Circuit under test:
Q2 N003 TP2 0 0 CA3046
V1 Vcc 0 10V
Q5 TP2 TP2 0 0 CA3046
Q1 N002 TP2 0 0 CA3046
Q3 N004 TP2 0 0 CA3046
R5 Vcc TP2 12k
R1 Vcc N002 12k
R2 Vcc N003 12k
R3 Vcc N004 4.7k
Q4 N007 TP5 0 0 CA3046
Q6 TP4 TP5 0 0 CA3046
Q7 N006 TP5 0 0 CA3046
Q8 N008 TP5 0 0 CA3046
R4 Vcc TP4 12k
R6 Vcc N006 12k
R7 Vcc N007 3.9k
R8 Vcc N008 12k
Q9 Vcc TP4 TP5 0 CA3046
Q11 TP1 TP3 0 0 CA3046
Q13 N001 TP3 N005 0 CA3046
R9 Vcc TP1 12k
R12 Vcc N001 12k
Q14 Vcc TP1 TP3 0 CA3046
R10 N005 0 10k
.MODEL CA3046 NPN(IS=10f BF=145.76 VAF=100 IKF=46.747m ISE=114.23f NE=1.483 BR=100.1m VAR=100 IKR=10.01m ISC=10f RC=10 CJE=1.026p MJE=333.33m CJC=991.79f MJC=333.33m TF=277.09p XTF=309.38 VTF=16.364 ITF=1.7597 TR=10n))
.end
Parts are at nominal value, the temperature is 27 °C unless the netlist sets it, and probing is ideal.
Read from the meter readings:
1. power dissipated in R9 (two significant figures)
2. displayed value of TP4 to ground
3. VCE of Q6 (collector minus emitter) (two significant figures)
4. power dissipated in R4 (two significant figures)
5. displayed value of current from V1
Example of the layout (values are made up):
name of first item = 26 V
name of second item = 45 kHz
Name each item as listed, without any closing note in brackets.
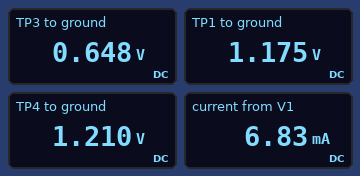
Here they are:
power dissipated in R9 = 6.5 mW
displayed value of TP4 to ground = 1.210 V
VCE of Q6 (collector minus emitter) = 1.2 V
power dissipated in R4 = 6.4 mW
displayed value of current from V1 = 6.83 mA
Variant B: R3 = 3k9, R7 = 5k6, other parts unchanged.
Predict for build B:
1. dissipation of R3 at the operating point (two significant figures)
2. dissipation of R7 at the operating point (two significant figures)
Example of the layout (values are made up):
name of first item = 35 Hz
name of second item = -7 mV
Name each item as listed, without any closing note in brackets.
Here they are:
dissipation of R3 at the operating point = 2.5 mW
dissipation of R7 at the operating point = 3.3 mW
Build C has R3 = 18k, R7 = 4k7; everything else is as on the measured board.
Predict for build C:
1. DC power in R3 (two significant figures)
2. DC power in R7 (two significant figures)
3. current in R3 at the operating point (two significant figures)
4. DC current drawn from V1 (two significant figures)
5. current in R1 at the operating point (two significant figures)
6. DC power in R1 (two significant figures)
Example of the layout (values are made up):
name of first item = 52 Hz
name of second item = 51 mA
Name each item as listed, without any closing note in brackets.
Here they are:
DC power in R3 = 5.4 mW
DC power in R7 = 2.8 mW
current in R3 at the operating point = 550 µA
DC current drawn from V1 = 6.4 mA
current in R1 at the operating point = 670 µA
DC power in R1 = 5.3 mW
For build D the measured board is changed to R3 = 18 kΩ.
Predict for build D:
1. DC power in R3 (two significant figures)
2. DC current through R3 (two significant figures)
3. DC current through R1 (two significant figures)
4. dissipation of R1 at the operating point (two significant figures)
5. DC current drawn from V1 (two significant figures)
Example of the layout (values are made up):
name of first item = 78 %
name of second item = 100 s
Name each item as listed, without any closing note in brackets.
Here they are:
DC power in R3 = 5.4 mW
DC current through R3 = 550 µA
DC current through R1 = 670 µA
dissipation of R1 at the operating point = 5.3 mW
DC current drawn from V1 = 6.4 mA
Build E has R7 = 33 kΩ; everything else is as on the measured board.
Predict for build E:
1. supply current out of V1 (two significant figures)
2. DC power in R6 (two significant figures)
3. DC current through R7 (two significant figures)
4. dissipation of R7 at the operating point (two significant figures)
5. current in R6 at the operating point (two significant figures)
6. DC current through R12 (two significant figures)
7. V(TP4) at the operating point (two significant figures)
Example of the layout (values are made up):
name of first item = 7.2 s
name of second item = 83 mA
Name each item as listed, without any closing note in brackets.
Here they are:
supply current out of V1 = 6.7 mA
DC power in R6 = 6.3 mW
DC current through R7 = 300 µA
dissipation of R7 at the operating point = 3.0 mW
current in R6 at the operating point = 720 µA
DC current through R12 = 11 µA
V(TP4) at the operating point = 1.3 V
